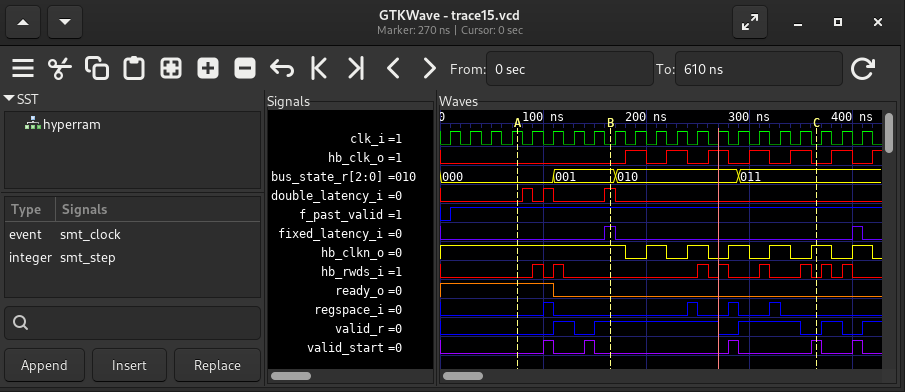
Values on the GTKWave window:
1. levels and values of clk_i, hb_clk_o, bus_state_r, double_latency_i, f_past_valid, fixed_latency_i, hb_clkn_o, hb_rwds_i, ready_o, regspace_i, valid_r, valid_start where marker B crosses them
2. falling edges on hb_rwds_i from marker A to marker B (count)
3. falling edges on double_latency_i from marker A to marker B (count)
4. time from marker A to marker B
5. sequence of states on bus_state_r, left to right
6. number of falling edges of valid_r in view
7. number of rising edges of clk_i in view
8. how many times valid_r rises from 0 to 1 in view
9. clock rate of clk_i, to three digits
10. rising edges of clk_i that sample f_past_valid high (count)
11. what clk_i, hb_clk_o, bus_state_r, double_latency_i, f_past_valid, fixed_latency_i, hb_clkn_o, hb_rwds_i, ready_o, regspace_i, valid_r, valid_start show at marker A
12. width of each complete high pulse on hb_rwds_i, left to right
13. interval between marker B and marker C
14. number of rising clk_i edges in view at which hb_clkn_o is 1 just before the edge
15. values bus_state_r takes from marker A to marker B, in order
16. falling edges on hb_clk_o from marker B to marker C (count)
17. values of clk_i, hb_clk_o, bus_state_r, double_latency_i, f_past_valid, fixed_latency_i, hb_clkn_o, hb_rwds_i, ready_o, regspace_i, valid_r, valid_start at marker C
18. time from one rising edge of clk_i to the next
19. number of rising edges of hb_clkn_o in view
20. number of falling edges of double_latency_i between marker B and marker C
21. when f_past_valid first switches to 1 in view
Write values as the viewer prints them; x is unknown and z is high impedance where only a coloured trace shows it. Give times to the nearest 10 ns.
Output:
clk_i=0, hb_clk_o=0, bus_state_r=001, double_latency_i=1, f_past_valid=1, fixed_latency_i=1, hb_clkn_o=1, hb_rwds_i=0, ready_o=0, regspace_i=0, valid_r=1, valid_start=0
2
2
90 ns
000, 001, 010, 011
4
21
5
50.0 MHz
20
clk_i=1, hb_clk_o=0, bus_state_r=000, double_latency_i=0, f_past_valid=1, fixed_latency_i=0, hb_clkn_o=1, hb_rwds_i=0, ready_o=1, regspace_i=0, valid_r=0, valid_start=0
10 ns, 10 ns, 10 ns, 10 ns, 10 ns, 10 ns, 10 ns, 10 ns
200 ns
15
000, 001
5
clk_i=0, hb_clk_o=0, bus_state_r=011, double_latency_i=0, f_past_valid=1, fixed_latency_i=0, hb_clkn_o=1, hb_rwds_i=0, ready_o=0, regspace_i=0, valid_r=0, valid_start=1
20 ns
6
1
10 ns
